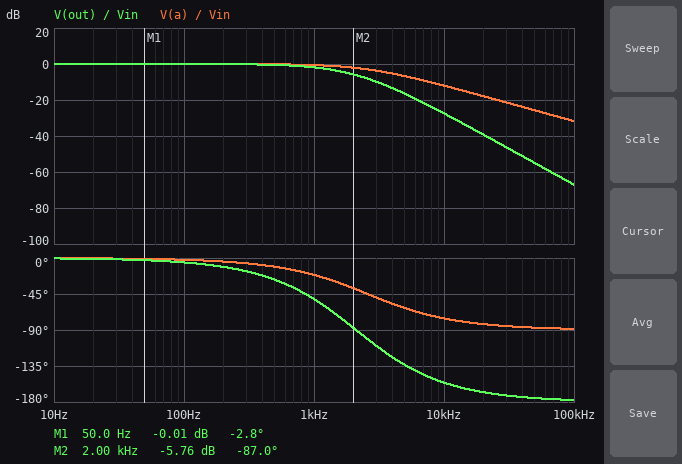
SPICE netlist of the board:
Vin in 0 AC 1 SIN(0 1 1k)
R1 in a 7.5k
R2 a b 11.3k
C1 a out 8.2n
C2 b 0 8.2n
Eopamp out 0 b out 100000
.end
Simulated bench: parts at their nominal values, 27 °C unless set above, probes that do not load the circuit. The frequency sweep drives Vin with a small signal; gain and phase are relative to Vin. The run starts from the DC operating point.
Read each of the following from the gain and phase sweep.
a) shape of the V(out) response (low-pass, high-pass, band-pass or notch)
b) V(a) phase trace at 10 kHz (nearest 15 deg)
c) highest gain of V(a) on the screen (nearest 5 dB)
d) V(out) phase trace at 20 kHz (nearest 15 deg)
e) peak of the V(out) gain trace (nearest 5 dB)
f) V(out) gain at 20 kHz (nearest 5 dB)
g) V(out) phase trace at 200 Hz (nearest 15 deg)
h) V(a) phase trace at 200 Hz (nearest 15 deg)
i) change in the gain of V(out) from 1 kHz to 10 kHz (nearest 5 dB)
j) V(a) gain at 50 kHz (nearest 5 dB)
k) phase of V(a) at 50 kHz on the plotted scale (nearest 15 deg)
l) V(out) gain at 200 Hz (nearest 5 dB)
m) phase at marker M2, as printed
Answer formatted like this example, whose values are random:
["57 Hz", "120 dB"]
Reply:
["low-pass", "-75 deg", "0 dB", "-165 deg", "0 dB", "-40 dB", "-15 deg", "0 deg", "-25 dB", "-25 dB", "-90 deg", "0 dB", "-87.0 deg"]
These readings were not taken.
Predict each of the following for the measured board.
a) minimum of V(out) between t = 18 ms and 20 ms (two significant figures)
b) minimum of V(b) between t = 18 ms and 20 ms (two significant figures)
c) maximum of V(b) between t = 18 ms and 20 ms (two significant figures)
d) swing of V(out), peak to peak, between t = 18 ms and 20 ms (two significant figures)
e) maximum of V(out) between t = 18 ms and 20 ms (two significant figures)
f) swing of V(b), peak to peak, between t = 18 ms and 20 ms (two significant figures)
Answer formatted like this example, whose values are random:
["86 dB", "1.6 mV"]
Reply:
["-810 mV", "-810 mV", "810 mV", "1.6 V", "810 mV", "1.6 V"]
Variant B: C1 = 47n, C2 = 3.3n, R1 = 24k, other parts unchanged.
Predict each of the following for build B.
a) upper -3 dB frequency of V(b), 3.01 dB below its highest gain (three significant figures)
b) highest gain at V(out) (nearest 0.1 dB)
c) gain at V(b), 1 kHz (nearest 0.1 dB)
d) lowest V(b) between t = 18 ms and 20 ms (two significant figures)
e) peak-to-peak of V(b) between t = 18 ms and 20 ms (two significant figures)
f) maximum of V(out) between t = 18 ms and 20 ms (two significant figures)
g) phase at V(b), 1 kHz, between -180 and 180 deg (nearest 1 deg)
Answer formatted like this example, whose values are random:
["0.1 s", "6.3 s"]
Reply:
["913 Hz", "5.3 dB", "0.1 dB", "-1.0 V", "2.0 V", "1.0 V", "-132 deg"]
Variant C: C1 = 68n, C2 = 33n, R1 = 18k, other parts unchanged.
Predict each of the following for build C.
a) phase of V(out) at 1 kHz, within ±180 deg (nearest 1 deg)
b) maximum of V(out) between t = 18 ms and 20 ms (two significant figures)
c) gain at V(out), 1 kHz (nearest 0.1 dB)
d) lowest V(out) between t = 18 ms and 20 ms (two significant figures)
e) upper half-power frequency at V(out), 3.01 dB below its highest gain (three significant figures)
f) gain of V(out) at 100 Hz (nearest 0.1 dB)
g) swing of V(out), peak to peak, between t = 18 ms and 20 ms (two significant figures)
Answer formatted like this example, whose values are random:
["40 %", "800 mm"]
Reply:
["-160 deg", "55 mV", "-25.1 dB", "-55 mV", "233 Hz", "-0.2 dB", "110 mV"]
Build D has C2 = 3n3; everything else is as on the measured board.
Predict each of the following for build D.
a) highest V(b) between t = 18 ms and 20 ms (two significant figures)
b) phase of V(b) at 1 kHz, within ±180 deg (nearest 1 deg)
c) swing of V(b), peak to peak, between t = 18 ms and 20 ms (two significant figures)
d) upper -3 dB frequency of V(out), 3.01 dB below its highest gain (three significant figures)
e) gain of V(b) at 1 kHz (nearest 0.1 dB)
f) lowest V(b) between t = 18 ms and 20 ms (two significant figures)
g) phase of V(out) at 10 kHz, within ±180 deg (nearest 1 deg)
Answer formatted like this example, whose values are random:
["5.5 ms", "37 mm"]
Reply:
["1.0 V", "-23 deg", "2.0 V", "3.56 kHz", "0.1 dB", "-1.0 V", "-154 deg"]
